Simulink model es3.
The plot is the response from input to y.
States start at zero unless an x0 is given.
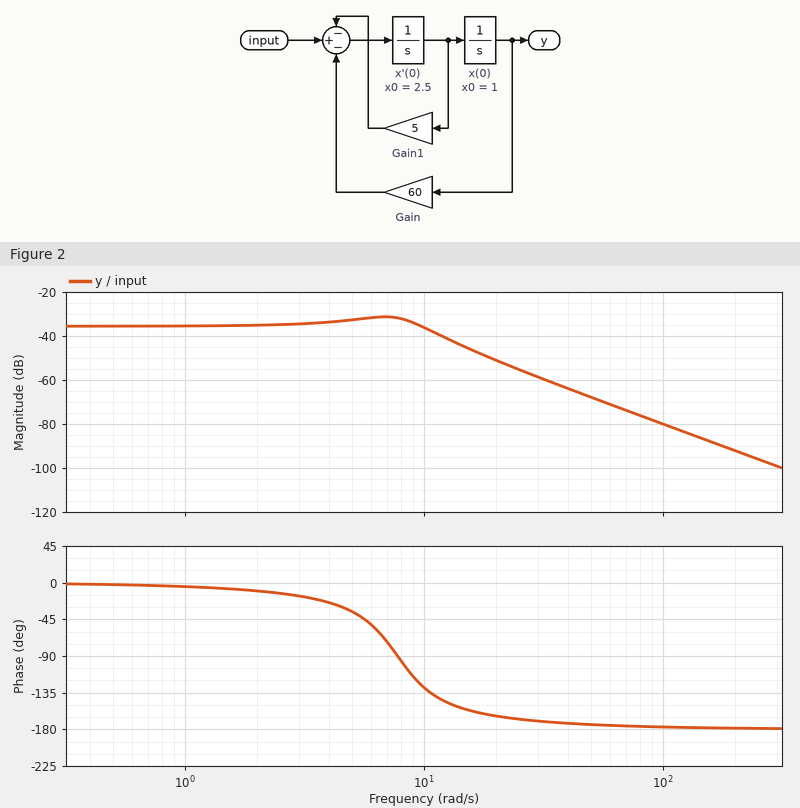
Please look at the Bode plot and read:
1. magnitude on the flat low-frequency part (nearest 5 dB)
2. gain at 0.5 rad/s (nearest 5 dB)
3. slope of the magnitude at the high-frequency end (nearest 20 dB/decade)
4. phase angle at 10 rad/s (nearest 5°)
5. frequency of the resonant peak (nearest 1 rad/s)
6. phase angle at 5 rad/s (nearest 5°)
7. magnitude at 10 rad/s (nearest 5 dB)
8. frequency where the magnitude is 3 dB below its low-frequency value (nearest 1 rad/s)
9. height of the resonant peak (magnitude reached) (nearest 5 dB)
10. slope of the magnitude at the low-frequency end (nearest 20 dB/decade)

-35 dB
-35 dB
-40 dB/decade
-130°
7 rad/s
-35°
-35 dB
11 rad/s
-30 dB
0 dB/decade
